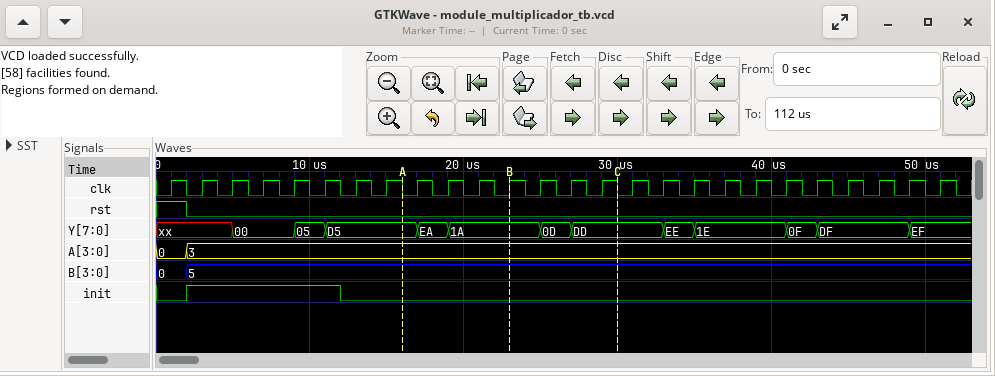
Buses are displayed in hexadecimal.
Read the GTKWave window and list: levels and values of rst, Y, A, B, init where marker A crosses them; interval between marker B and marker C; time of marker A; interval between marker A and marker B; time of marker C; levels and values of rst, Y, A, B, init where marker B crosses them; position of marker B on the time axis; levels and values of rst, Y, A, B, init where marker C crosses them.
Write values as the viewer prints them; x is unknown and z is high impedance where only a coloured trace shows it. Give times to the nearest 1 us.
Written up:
rst=0, Y=D5, A=3, B=5, init=0
7 us
16 us
7 us
30 us
rst=0, Y=1A, A=3, B=5, init=0
23 us
rst=0, Y=DD, A=3, B=5, init=0
